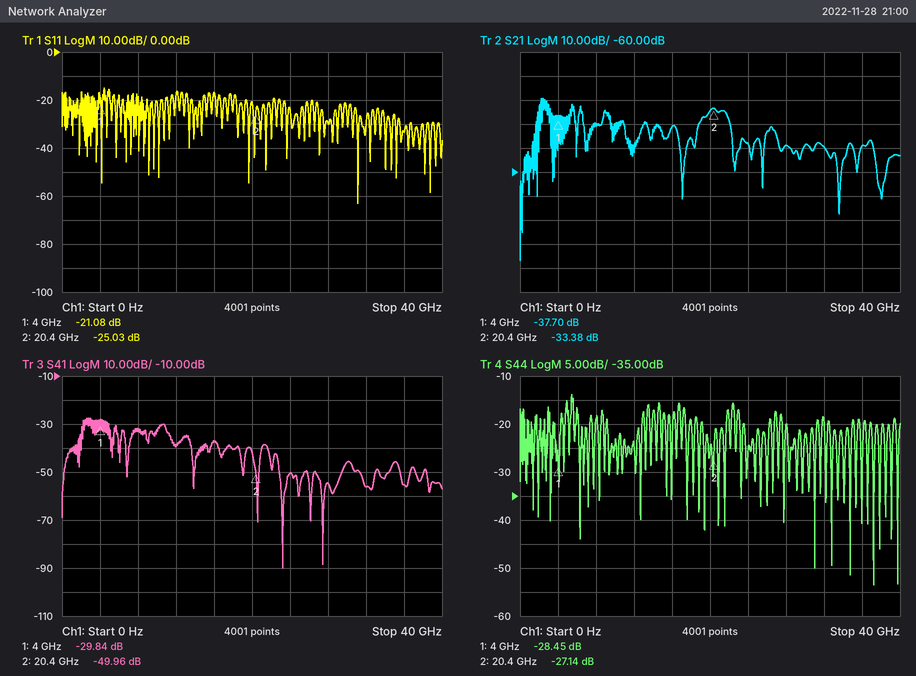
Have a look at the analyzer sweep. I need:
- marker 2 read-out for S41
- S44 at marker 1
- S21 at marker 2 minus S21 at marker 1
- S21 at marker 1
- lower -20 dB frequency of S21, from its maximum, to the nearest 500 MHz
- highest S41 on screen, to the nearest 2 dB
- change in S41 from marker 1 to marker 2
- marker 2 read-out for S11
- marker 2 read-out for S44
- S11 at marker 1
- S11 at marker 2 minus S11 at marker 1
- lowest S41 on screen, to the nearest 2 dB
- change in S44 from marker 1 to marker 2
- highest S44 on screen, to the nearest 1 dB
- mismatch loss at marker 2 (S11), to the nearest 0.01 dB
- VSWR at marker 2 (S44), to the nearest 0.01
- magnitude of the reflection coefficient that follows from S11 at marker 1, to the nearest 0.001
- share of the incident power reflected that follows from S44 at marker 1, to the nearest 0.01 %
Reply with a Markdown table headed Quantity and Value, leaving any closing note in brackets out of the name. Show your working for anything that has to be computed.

| Quantity | Value |
|---|---|
| marker 2 read-out for S41 | -49.96 dB |
| S44 at marker 1 | -28.45 dB |
| S21 at marker 2 minus S21 at marker 1 | -33.38 − (-37.7) = 4.32 dB |
| S21 at marker 1 | -37.70 dB |
| lower -20 dB frequency of S21, from its maximum, to the nearest 500 MHz | 2.0 GHz |
| highest S41 on screen, to the nearest 2 dB | -28 dB |
| change in S41 from marker 1 to marker 2 | -49.96 − (-29.84) = -20.12 dB |
| marker 2 read-out for S11 | -25.03 dB |
| marker 2 read-out for S44 | -27.14 dB |
| S11 at marker 1 | -21.08 dB |
| S11 at marker 2 minus S11 at marker 1 | -25.03 − (-21.08) = -3.95 dB |
| lowest S41 on screen, to the nearest 2 dB | -90 dB |
| change in S44 from marker 1 to marker 2 | -27.14 − (-28.45) = 1.31 dB |
| highest S44 on screen, to the nearest 1 dB | -14 dB |
| mismatch loss at marker 2 (S11), to the nearest 0.01 dB | −10 log10(1 − 10^(-25.03/10)) ≈ 0.01 dB |
| VSWR at marker 2 (S44), to the nearest 0.01 | (1 + 0.0440)/(1 − 0.0440) ≈ 1.09 |
| magnitude of the reflection coefficient that follows from S11 at marker 1, to the nearest 0.001 | 10^(-21.08/20) ≈ 0.088 |
| share of the incident power reflected that follows from S44 at marker 1, to the nearest 0.01 % | 10^(-28.45/10) ≈ 0.14 % |
